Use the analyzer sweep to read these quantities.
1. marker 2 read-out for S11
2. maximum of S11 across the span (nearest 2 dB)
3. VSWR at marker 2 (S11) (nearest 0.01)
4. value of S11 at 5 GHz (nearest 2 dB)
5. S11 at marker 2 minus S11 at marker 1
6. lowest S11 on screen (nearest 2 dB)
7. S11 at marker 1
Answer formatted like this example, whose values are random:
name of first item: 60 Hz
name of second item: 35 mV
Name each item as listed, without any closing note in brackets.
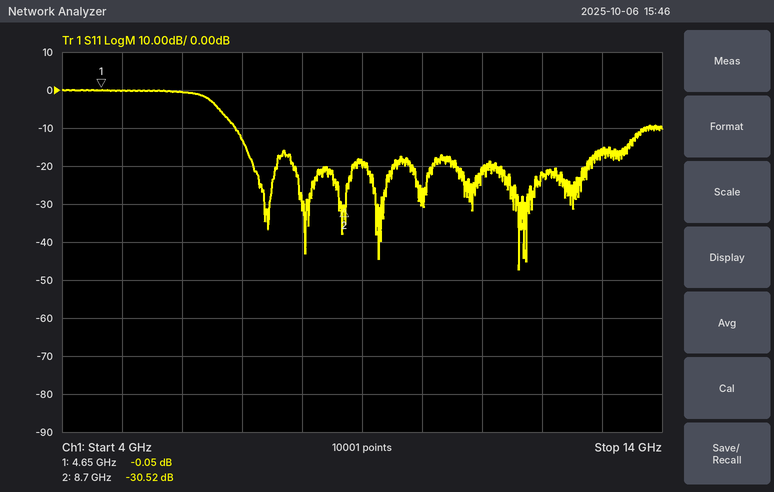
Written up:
marker 2 read-out for S11: -30.52 dB
maximum of S11 across the span: 0 dB
VSWR at marker 2 (S11): 1.06
value of S11 at 5 GHz: 0 dB
S11 at marker 2 minus S11 at marker 1: -30.47 dB
lowest S11 on screen: -48 dB
S11 at marker 1: -0.05 dB
